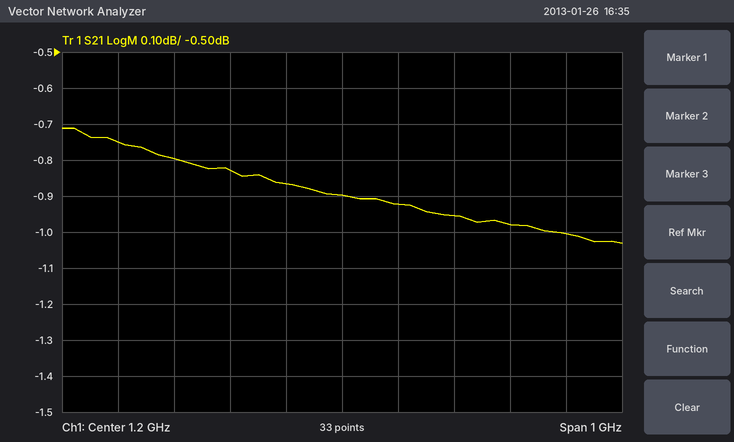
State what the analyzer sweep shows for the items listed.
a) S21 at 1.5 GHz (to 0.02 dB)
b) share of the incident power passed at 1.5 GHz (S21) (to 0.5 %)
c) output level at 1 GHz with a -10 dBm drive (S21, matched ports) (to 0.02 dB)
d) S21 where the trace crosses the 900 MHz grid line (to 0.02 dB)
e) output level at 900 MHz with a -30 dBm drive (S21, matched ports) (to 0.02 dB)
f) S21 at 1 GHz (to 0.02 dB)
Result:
-0.98 dB
80.0 %
-10.82 dBm
-0.80 dB
-30.80 dBm
-0.82 dB
